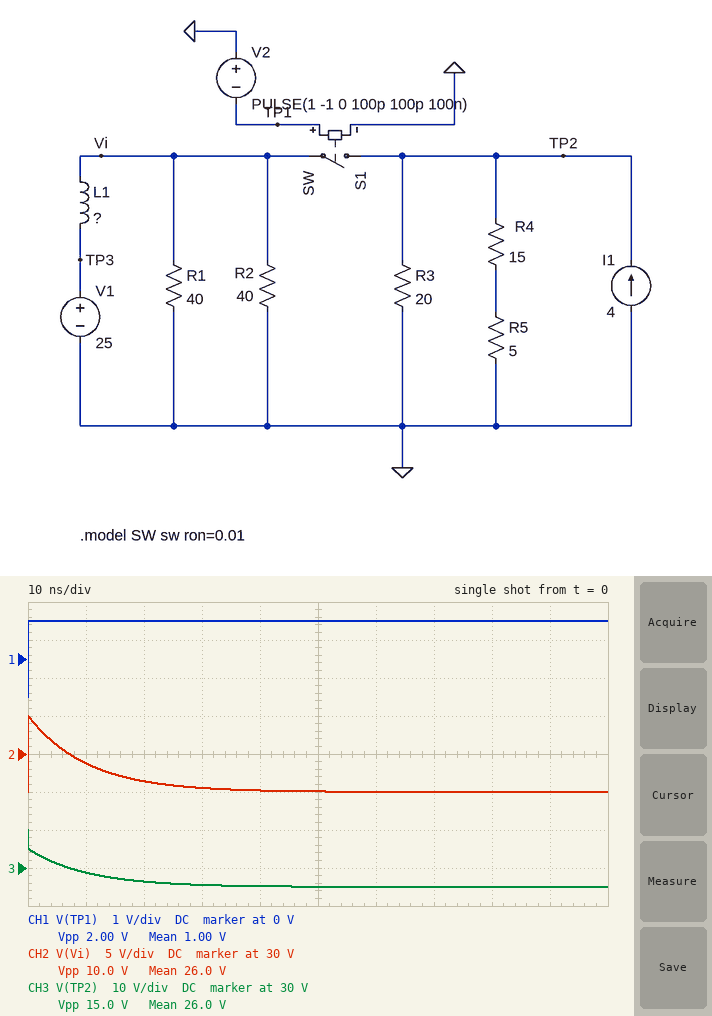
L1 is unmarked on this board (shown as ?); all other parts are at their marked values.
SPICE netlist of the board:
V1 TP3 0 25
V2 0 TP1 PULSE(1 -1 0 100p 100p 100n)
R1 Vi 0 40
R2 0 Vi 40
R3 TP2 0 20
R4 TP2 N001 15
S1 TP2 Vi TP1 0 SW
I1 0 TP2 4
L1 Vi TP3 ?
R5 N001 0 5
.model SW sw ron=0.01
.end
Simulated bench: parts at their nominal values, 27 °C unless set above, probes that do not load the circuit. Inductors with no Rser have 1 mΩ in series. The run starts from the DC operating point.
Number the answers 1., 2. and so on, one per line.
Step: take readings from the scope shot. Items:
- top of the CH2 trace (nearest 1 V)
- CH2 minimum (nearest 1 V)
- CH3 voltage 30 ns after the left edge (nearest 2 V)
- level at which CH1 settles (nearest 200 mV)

1. 35 V
2. 25 V
3. 26 V
4. 1.0 V
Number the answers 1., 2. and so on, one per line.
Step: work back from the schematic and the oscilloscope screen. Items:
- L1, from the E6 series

1. 68 nH
